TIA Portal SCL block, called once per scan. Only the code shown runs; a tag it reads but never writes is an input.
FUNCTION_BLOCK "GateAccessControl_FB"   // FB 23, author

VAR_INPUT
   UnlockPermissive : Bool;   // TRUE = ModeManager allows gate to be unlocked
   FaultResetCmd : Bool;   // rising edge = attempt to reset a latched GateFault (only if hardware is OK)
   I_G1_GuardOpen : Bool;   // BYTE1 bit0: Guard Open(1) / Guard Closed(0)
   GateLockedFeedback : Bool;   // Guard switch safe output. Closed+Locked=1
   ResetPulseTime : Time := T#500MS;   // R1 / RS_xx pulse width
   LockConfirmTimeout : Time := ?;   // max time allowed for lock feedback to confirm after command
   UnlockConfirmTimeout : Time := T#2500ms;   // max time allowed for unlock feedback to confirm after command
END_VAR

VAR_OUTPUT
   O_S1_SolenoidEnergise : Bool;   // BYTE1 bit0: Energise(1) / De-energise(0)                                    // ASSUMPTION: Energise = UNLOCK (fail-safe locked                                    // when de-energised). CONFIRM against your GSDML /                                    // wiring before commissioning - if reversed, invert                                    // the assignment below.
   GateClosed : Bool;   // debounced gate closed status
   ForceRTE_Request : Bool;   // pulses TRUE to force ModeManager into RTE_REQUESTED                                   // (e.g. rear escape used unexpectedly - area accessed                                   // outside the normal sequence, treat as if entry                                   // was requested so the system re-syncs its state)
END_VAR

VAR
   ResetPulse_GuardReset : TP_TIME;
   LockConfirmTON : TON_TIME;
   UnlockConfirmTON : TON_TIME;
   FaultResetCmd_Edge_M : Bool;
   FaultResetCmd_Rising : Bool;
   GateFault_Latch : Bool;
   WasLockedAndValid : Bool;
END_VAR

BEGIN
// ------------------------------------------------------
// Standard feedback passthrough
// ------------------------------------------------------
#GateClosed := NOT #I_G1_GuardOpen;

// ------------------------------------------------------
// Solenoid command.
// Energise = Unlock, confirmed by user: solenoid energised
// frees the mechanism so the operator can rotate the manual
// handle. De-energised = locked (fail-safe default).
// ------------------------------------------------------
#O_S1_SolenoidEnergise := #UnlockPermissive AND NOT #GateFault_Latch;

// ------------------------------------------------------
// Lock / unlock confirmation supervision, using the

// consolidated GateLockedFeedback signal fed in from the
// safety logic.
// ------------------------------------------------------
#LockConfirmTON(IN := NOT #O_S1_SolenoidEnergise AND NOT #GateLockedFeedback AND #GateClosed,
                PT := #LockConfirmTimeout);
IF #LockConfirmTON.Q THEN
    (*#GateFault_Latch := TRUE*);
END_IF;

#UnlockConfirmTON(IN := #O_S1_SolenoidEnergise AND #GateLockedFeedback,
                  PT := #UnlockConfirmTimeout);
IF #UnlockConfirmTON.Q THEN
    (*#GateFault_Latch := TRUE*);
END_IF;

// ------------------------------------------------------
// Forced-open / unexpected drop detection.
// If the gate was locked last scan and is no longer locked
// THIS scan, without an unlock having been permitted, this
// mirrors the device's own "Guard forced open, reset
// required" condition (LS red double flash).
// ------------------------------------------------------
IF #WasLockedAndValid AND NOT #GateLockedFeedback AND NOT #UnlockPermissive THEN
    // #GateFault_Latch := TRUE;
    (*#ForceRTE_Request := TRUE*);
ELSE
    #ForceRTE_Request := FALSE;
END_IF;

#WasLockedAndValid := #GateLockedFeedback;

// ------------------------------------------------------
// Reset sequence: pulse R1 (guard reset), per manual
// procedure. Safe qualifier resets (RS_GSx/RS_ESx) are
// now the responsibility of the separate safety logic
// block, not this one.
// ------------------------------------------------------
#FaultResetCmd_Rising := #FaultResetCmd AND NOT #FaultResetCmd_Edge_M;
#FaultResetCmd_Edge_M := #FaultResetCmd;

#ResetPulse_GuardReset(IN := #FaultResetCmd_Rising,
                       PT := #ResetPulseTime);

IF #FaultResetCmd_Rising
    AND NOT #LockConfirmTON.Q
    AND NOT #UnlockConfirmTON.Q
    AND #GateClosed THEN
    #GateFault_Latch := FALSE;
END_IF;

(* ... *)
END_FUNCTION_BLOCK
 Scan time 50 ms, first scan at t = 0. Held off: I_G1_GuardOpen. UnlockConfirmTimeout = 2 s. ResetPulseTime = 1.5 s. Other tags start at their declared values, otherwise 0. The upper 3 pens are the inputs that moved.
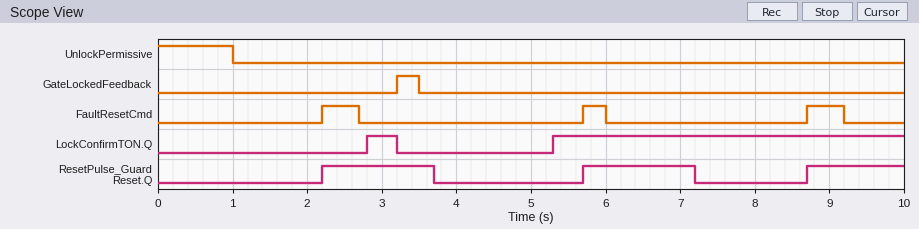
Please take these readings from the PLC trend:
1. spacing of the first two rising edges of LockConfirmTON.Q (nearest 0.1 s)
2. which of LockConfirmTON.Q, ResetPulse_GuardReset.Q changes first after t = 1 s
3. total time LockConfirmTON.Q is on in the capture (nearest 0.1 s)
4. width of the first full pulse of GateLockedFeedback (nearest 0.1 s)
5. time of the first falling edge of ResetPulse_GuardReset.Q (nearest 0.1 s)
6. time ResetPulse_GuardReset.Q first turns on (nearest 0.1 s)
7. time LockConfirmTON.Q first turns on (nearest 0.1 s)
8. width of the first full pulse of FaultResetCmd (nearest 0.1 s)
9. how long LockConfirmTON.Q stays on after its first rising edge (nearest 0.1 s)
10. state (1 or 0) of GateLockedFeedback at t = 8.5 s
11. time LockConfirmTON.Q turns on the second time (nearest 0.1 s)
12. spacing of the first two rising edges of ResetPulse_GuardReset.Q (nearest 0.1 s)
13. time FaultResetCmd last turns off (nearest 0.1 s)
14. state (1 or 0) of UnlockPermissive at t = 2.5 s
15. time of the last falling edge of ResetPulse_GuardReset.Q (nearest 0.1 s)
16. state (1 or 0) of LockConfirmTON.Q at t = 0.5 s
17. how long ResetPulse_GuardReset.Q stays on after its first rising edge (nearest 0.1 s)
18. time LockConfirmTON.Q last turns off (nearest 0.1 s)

2.5 s
ResetPulse_GuardReset.Q
5.1 s
0.3 s
3.7 s
2.2 s
2.8 s
0.5 s
0.4 s
0
5.3 s
3.5 s
9.2 s
0
7.2 s
0
1.5 s
3.2 s
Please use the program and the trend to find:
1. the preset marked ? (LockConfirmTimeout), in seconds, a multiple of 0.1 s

1.8 s
